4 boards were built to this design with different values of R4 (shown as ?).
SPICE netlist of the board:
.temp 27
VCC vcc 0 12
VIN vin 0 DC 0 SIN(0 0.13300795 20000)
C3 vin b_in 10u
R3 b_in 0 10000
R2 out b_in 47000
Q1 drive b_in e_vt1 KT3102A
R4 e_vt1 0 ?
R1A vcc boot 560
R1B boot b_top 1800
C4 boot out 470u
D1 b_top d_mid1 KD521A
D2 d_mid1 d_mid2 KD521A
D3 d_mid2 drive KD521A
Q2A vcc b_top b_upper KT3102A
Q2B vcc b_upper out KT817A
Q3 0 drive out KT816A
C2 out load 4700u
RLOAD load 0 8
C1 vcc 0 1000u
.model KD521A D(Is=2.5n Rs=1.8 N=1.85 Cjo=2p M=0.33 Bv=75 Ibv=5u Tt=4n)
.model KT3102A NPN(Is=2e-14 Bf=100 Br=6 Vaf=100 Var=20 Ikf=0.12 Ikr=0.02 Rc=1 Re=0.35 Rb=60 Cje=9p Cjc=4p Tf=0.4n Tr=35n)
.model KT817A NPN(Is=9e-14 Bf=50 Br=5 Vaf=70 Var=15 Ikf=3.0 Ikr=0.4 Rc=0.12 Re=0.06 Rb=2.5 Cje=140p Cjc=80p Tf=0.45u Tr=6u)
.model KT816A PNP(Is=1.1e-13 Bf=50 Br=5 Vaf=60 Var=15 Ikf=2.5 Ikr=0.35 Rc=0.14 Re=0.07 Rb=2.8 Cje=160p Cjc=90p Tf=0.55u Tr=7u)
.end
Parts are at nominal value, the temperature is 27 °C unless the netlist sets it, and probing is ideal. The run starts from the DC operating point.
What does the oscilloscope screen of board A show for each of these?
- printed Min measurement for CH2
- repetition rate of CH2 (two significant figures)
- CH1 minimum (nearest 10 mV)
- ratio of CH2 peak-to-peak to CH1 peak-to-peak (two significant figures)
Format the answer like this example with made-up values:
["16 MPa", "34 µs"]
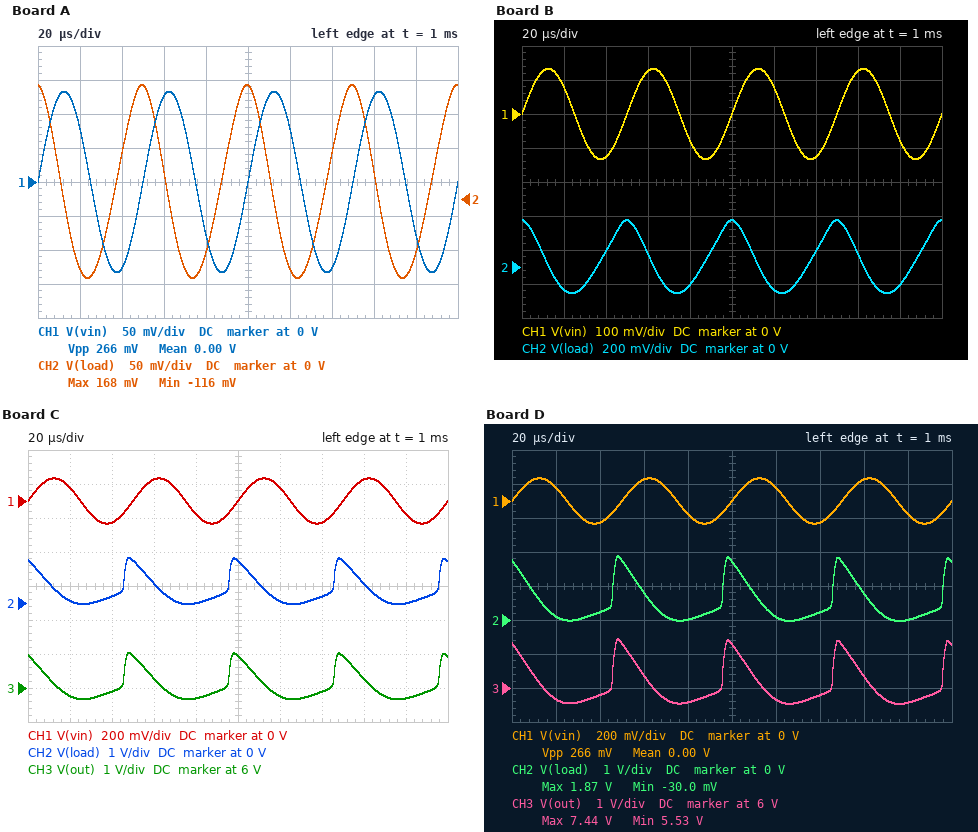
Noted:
["-116 mV", "20 kHz", "-130 mV", "1.1"]
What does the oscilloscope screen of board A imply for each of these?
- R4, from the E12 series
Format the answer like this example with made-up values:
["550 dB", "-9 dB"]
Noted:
["120 Ω"]
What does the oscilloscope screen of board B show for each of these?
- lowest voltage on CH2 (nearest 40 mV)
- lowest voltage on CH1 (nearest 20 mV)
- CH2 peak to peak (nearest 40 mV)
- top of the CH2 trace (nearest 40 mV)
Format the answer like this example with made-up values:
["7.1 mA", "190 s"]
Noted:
["-160 mV", "-140 mV", "440 mV", "280 mV"]
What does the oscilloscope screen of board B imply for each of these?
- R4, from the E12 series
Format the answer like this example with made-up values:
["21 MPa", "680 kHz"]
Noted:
["82 Ω"]
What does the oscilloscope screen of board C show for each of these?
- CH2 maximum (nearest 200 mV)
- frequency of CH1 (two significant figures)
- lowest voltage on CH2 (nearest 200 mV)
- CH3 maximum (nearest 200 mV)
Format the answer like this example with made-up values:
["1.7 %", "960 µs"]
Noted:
["1.4 V", "20 kHz", "0 V", "7.0 V"]
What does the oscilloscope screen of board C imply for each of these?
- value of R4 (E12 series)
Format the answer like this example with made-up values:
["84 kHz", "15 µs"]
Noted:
["47 Ω"]
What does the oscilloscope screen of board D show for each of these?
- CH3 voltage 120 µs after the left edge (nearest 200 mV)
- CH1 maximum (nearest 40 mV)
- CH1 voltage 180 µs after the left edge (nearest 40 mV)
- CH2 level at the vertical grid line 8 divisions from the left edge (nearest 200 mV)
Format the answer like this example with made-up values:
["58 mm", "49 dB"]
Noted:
["5.6 V", "120 mV", "-80 mV", "800 mV"]
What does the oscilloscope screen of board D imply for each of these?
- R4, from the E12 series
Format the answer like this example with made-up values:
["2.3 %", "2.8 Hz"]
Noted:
["33 Ω"]
